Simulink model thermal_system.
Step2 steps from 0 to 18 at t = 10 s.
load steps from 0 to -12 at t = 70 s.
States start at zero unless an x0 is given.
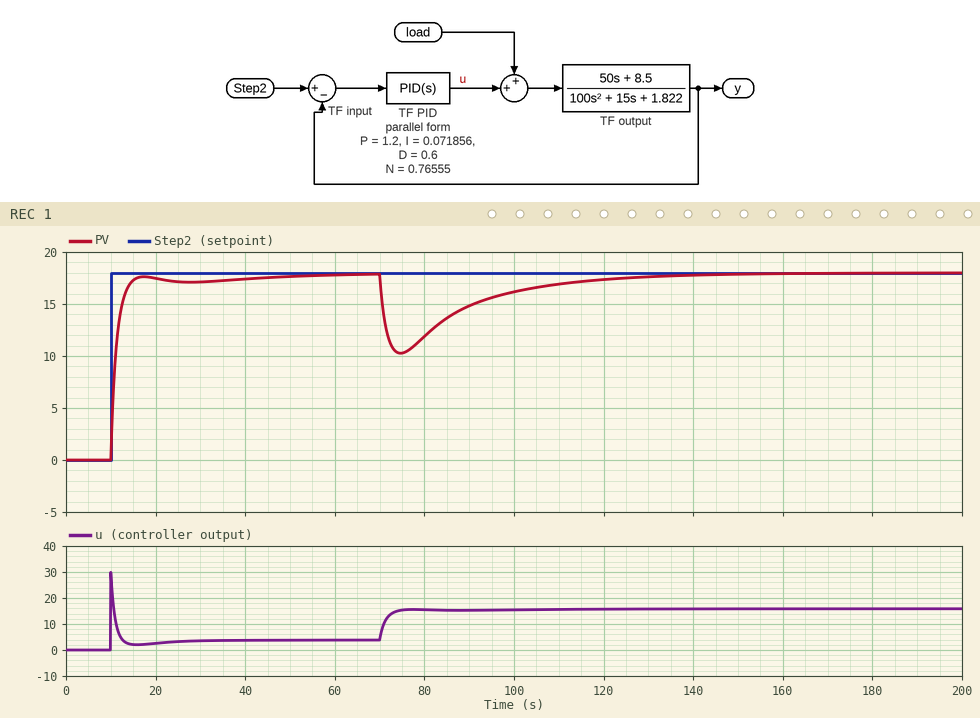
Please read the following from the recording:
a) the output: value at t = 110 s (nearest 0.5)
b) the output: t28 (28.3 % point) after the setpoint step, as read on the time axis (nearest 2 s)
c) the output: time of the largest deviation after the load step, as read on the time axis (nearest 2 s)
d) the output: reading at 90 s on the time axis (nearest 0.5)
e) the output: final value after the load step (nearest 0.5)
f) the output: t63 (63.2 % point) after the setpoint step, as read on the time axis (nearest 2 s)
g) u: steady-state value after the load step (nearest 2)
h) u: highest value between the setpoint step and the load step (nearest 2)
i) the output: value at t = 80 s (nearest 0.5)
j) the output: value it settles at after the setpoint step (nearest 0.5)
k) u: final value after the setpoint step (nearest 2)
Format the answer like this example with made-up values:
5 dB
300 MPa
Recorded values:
17.0
10 s
74 s
15.0
18.0
12 s
16
30
12.0
18.0
4
